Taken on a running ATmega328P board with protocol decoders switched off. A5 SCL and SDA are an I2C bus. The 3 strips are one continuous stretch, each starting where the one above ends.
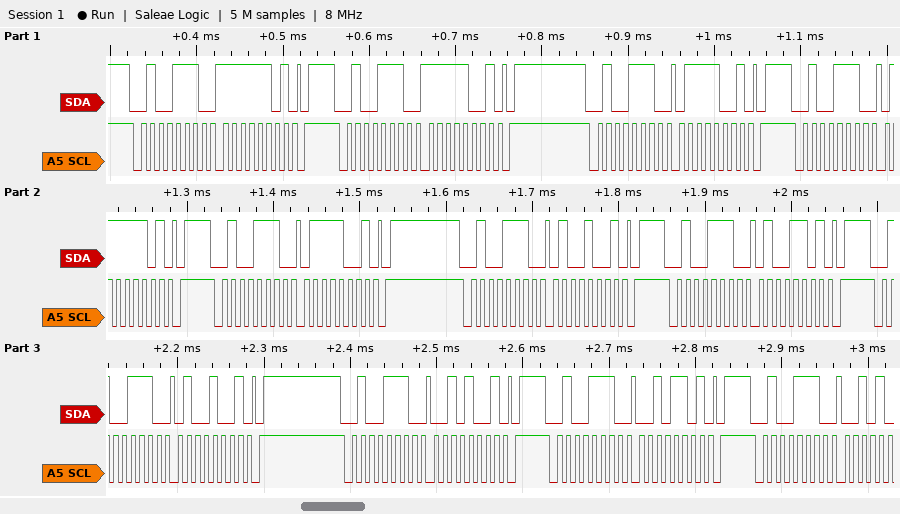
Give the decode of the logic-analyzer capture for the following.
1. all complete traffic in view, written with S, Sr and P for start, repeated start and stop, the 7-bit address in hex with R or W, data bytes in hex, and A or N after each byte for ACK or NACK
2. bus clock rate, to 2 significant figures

S 27W A FD A P S 27W A F9 A P S 27W A 79 A P S 27W A 7D A P S 27W A 79 A P S 27W A 49 A P S 27W A 4D A P S 27W A 49 A P S 27W A 29 A P S 27W A 2D A P S 27W A
100 kHz
